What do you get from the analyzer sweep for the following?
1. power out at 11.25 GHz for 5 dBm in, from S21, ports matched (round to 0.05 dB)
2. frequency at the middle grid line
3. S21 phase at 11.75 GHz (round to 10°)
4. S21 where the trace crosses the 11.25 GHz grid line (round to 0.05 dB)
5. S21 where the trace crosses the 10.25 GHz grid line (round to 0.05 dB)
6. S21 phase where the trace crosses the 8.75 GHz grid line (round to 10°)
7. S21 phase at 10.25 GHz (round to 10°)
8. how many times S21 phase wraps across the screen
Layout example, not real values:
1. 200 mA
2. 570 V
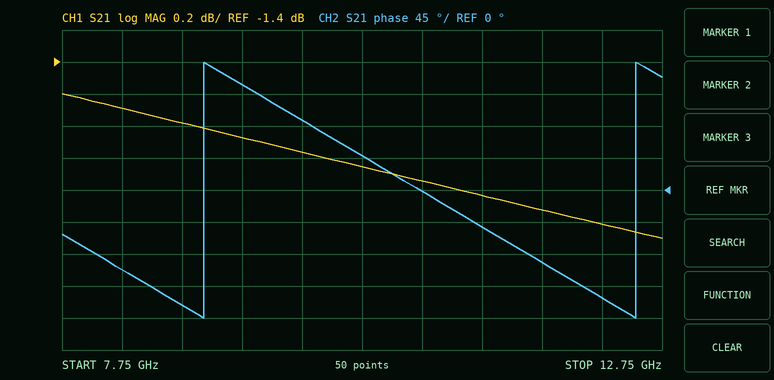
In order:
1. 2.75 dBm
2. 10.25 GHz
3. -100°
4. -2.25 dB
5. -2.05 dB
6. -160°
7. 50°
8. 2
